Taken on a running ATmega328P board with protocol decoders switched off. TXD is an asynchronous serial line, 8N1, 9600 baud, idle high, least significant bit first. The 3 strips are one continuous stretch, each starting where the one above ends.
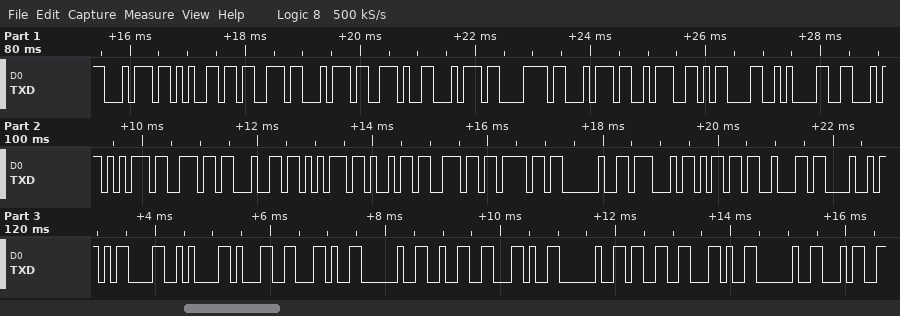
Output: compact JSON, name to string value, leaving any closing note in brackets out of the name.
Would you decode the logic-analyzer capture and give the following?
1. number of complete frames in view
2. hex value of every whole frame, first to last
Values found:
{"number of complete frames in view": "36", "hex value of every whole frame, first to last": "0x74 0x65 0x73 0x74 0x2E 0x74 0x78 0x74 0x3A 0x0D 0x0A 0x46 0x75 0x6E 0x64 0x75 0x69 0x6E 0x6F 0x20 0x47 0x6D 0x62 0x48 0x0D 0x0A 0x31 0x2C 0x20 0x32 0x2C 0x20 0x33 0x2C 0x20 0x34"}
